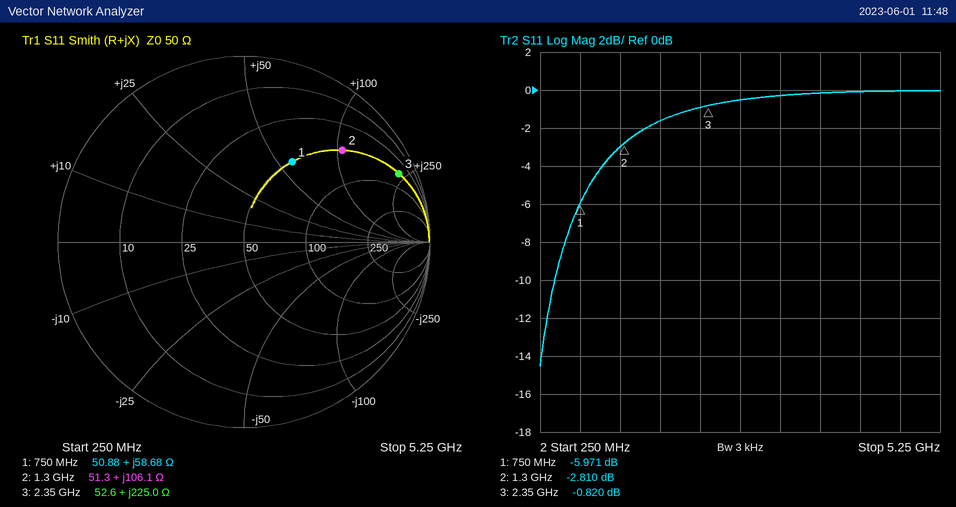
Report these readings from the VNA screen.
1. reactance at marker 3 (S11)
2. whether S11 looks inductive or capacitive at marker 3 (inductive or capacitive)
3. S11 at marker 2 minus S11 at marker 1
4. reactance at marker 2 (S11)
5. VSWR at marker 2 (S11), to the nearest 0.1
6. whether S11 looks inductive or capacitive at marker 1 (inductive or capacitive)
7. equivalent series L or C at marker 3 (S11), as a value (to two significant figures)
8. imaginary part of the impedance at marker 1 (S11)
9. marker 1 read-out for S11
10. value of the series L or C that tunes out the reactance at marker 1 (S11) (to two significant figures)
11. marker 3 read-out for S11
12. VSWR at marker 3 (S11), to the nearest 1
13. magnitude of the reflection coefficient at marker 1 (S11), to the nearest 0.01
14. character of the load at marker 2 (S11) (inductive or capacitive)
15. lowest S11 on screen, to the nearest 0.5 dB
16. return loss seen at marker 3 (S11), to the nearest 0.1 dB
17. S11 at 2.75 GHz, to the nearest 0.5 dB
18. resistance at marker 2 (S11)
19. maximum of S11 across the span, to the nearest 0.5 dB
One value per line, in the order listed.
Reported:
+225.0 Ω
inductive
3.161 dB
+106.1 Ω
6.2
inductive
15 nH
+58.68 Ω
-5.971 dB
3.6 pF
-0.820 dB
21
0.50
inductive
-14.5 dB
0.8 dB
-0.5 dB
51.3 Ω
0.0 dB
